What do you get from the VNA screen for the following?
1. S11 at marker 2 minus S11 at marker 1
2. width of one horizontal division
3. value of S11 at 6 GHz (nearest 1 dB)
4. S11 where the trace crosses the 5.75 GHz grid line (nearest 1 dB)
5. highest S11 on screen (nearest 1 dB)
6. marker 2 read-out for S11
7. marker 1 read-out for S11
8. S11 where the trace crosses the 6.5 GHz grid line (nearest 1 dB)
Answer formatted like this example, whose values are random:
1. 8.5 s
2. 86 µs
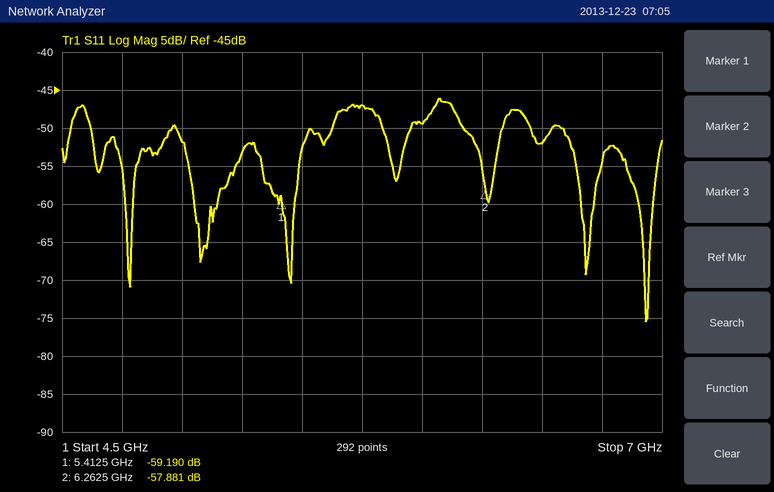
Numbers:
1. 1.309 dB
2. 250 MHz
3. -49 dB
4. -47 dB
5. -46 dB
6. -57.881 dB
7. -59.190 dB
8. -52 dB
